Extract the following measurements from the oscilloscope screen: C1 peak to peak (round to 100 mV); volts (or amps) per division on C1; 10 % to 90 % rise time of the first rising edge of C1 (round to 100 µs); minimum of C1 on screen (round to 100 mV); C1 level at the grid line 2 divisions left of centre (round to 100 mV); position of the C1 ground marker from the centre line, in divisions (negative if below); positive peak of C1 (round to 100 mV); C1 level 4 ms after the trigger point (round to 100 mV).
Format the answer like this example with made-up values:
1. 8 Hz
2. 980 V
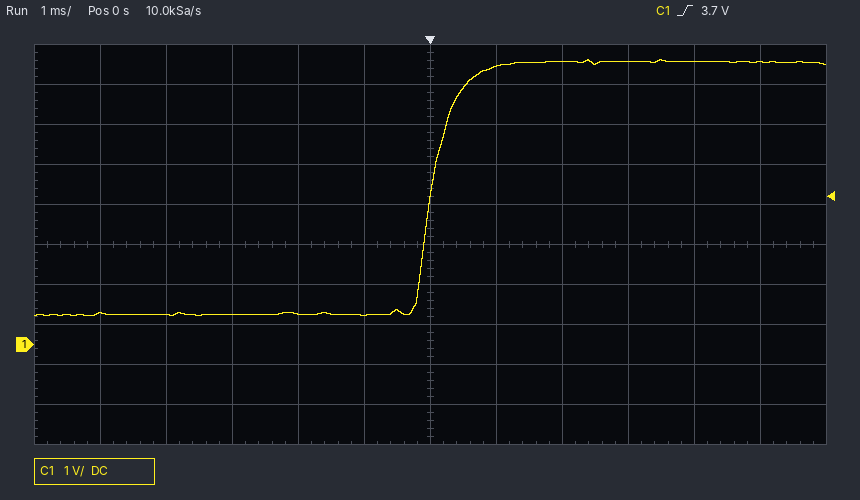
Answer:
1. 6.4 V
2. 1 V
3. 700 µs
4. 700 mV
5. 800 mV
6. -2.5 div
7. 7.1 V
8. 7.1 V
